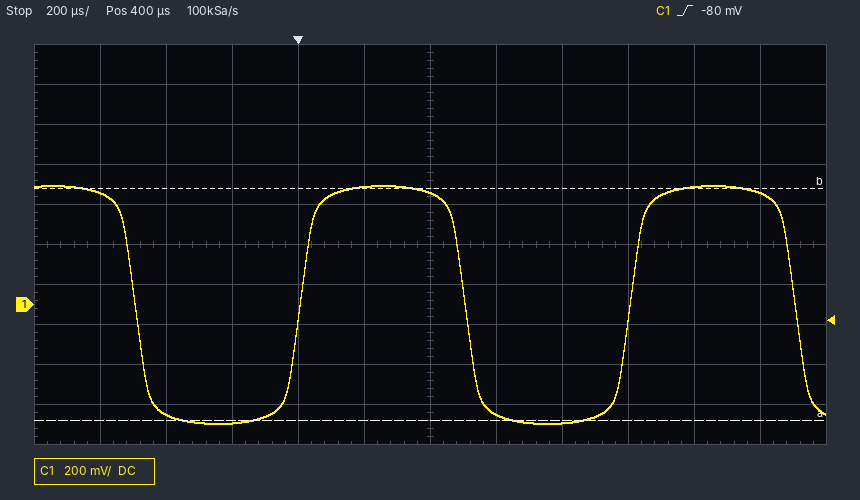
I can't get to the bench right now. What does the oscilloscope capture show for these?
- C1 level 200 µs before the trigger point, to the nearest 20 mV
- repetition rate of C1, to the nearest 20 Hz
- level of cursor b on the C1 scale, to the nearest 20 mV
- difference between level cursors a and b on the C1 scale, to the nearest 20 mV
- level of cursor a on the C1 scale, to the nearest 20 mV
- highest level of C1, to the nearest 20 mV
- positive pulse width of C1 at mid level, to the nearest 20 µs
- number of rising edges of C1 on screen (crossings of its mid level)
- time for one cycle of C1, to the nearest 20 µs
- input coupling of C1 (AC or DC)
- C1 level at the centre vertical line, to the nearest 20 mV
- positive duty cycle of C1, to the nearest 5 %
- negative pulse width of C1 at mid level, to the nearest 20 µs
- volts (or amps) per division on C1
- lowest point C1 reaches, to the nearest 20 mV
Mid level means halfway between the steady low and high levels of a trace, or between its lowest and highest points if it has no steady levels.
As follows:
-600 mV
1.00 kHz
580 mV
1.16 V
-580 mV
600 mV
500 µs
2
1.00 ms
DC
560 mV
50 %
500 µs
200 mV
-600 mV
